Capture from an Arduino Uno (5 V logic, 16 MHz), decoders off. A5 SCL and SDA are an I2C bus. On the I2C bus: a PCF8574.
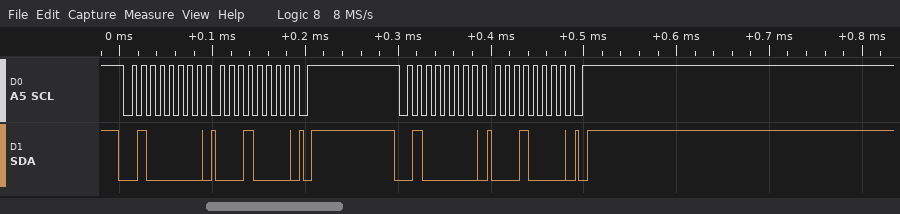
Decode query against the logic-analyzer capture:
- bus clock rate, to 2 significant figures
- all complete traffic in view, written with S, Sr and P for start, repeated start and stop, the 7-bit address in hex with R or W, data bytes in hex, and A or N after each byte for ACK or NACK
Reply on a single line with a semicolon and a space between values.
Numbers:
100 kHz; S 20W A 10 A P S 20W A 10 A P
